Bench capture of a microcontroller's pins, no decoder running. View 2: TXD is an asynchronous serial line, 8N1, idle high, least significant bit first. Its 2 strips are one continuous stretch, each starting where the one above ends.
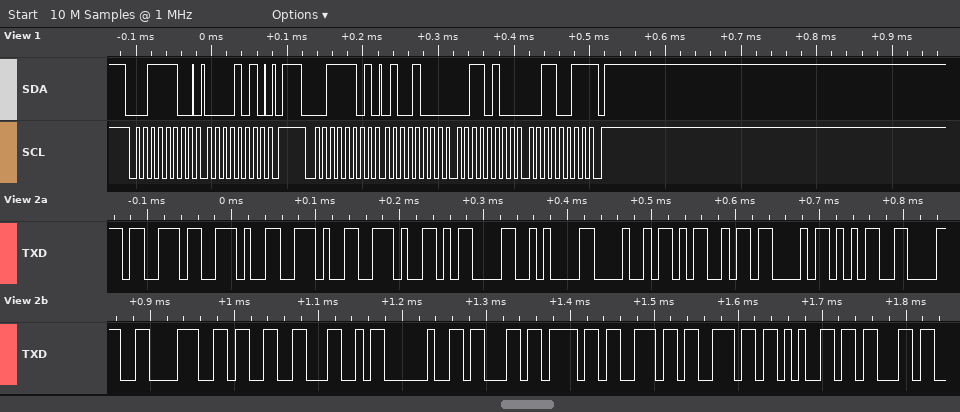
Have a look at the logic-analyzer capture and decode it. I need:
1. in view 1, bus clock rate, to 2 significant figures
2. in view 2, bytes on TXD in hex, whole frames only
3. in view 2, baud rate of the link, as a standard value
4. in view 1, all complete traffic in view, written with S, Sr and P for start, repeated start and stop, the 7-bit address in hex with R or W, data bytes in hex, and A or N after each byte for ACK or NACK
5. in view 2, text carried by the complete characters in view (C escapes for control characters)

100 kHz
73 2E 2E 2E 0D 0A 48 4D 43 35 38 38 33 4C 20 63 6F 6E 6E 65 63
115200 baud
S 1EW A 0A A P S 1ER A 48 A 34 A 33 N P
"s...\r\nHMC5883L connec"
